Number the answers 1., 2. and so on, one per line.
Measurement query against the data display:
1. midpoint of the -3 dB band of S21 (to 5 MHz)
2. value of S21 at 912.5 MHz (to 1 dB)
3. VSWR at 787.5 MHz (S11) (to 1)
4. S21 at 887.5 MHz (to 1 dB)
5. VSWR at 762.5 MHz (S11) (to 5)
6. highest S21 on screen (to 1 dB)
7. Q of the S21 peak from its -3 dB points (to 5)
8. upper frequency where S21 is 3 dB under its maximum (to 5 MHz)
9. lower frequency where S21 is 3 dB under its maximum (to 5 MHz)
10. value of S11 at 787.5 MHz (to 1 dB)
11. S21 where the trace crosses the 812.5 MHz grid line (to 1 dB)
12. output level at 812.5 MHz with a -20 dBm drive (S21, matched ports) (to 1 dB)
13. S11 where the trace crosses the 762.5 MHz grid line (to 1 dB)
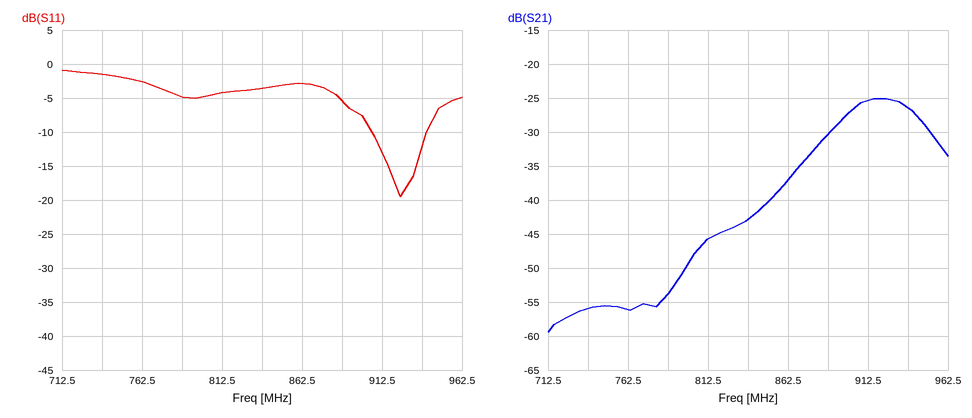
1. 920 MHz
2. -25 dB
3. 4
4. -30 dB
5. 5
6. -25 dB
7. 20
8. 945 MHz
9. 895 MHz
10. -5 dB
11. -46 dB
12. -66 dBm
13. -3 dB
